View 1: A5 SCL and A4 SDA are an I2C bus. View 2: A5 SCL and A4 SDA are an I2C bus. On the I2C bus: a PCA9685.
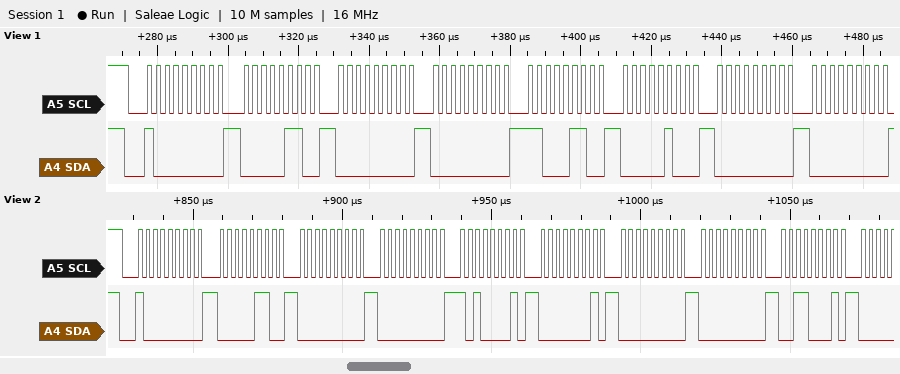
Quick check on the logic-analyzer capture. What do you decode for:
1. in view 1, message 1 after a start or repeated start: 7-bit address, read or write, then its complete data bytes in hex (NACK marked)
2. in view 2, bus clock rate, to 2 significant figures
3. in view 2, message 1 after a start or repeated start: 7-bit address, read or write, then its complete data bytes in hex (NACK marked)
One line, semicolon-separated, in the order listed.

0x40 write: 06 00 00 C6 04 00 00; 400 kHz; 0x40 write: 06 00 00 A1 01 00 00 31
